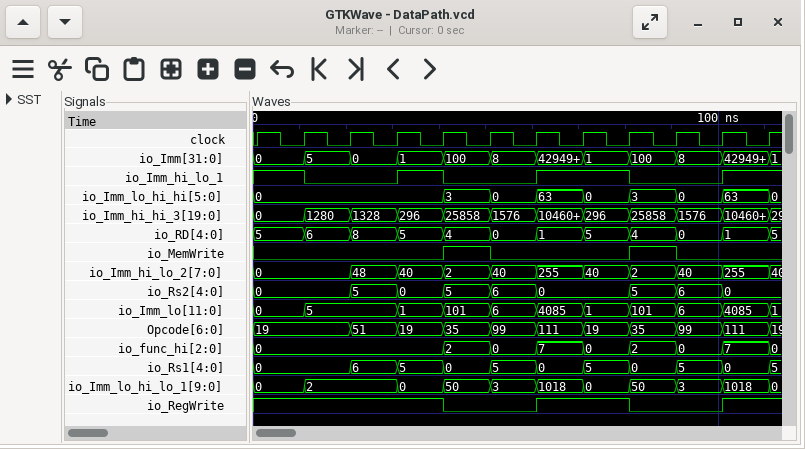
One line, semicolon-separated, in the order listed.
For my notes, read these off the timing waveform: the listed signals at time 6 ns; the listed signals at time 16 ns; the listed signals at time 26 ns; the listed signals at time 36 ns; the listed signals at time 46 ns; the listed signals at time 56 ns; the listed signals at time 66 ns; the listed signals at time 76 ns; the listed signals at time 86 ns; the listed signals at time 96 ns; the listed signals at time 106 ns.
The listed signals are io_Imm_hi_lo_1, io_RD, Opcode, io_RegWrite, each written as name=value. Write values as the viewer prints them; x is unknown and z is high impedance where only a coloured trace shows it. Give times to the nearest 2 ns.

io_Imm_hi_lo_1=1, io_RD=5, Opcode=19, io_RegWrite=1; io_Imm_hi_lo_1=0, io_RD=6, Opcode=19, io_RegWrite=1; io_Imm_hi_lo_1=0, io_RD=8, Opcode=51, io_RegWrite=1; io_Imm_hi_lo_1=1, io_RD=5, Opcode=19, io_RegWrite=1; io_Imm_hi_lo_1=0, io_RD=4, Opcode=35, io_RegWrite=0; io_Imm_hi_lo_1=0, io_RD=0, Opcode=99, io_RegWrite=0; io_Imm_hi_lo_1=1, io_RD=1, Opcode=111, io_RegWrite=1; io_Imm_hi_lo_1=1, io_RD=5, Opcode=19, io_RegWrite=1; io_Imm_hi_lo_1=0, io_RD=4, Opcode=35, io_RegWrite=0; io_Imm_hi_lo_1=0, io_RD=0, Opcode=99, io_RegWrite=0; io_Imm_hi_lo_1=1, io_RD=1, Opcode=111, io_RegWrite=1
